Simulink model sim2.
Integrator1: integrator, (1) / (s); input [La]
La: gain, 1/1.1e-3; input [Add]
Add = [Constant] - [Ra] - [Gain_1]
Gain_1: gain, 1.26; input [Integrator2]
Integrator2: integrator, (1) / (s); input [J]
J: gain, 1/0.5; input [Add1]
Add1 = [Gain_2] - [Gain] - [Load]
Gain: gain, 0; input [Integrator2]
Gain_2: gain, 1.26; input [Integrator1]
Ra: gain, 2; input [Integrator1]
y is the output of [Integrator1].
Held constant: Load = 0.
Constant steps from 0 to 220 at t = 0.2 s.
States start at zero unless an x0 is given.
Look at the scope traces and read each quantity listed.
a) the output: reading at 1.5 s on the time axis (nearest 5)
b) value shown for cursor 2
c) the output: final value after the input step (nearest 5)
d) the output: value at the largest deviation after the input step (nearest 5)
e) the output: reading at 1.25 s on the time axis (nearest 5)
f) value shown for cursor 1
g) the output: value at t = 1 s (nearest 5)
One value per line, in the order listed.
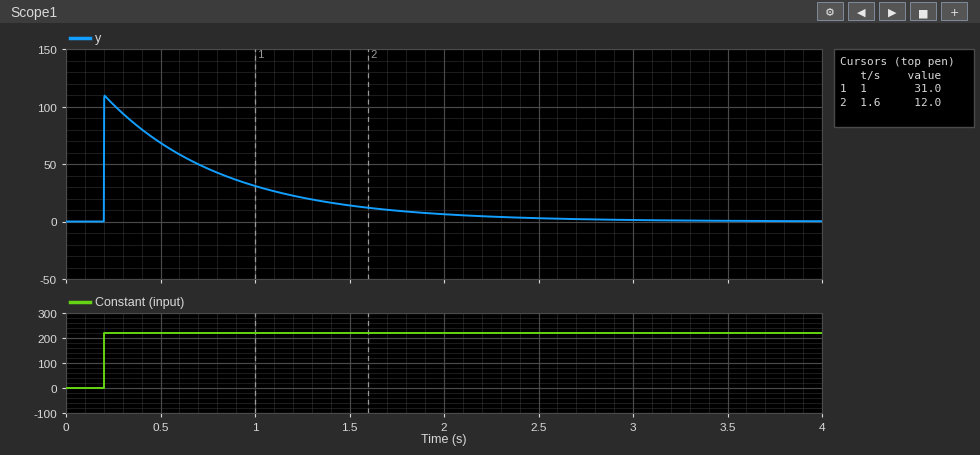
15
12.0
0
110
20
31.0
30
